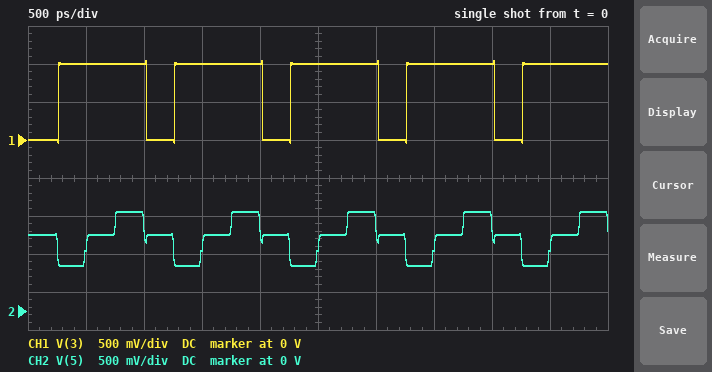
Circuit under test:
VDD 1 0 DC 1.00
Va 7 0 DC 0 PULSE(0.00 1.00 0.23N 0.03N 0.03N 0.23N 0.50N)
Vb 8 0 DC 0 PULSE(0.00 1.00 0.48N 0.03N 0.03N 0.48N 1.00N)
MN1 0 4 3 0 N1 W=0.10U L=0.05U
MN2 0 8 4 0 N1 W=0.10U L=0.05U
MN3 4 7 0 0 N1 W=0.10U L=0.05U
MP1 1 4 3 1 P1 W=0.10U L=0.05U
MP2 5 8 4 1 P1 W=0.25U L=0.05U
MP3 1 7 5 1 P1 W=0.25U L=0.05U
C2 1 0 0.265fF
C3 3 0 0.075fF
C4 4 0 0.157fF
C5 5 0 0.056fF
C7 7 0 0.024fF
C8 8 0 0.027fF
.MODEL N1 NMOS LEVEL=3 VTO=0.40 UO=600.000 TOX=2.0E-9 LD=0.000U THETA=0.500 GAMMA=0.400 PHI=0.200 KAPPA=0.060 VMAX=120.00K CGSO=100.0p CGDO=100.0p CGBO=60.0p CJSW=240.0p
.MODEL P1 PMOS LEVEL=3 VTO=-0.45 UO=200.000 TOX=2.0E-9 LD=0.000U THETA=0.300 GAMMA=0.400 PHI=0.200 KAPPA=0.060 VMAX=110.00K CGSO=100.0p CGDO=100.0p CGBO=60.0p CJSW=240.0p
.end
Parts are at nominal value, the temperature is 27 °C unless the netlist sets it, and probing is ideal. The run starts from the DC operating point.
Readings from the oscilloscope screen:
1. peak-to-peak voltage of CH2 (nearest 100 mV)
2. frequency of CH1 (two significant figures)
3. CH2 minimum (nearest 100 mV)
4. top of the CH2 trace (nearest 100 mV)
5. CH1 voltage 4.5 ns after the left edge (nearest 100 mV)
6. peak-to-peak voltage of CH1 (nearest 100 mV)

700 mV
1.0 GHz
600 mV
1.3 V
1.0 V
1.1 V
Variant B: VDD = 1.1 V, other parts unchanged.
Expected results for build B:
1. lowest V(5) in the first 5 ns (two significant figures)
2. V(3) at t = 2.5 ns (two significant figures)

610 mV
1.1 V
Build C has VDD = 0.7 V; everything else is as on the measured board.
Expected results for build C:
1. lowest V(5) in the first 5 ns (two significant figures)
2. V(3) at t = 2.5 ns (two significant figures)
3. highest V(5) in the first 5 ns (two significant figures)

520 mV
700 mV
1.1 V
